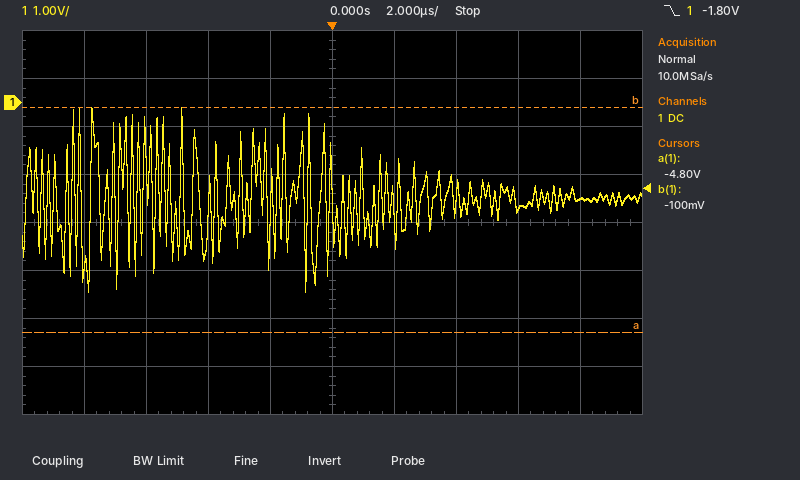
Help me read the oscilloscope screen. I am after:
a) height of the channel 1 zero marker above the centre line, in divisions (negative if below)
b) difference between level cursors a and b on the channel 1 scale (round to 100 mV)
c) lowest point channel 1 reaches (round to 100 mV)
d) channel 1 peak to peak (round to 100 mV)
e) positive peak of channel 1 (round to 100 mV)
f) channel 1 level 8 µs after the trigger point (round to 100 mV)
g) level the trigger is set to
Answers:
+2.5 div
4.7 V
-3.9 V
3.8 V
-100 mV
-2.0 V
-1.80 V
